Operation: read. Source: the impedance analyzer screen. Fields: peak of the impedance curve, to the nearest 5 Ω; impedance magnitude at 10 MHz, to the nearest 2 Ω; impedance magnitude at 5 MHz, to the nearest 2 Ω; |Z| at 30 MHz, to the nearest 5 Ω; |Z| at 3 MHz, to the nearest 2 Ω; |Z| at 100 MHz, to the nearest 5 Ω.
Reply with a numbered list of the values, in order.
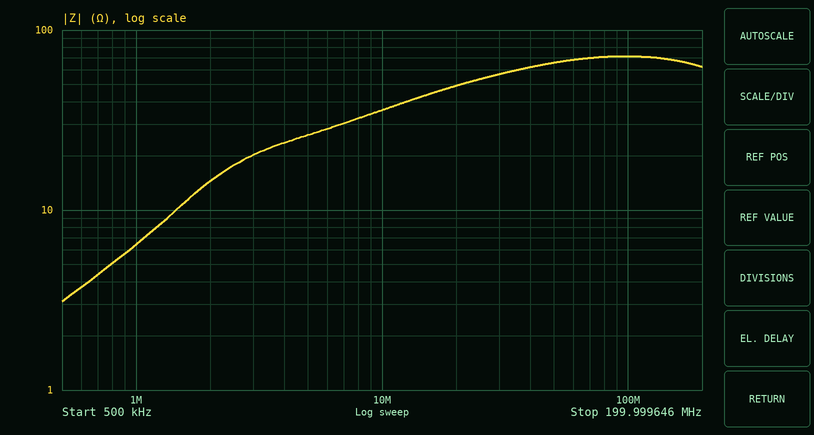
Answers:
1. 70 Ω
2. 36 Ω
3. 26 Ω
4. 55 Ω
5. 20 Ω
6. 70 Ω
